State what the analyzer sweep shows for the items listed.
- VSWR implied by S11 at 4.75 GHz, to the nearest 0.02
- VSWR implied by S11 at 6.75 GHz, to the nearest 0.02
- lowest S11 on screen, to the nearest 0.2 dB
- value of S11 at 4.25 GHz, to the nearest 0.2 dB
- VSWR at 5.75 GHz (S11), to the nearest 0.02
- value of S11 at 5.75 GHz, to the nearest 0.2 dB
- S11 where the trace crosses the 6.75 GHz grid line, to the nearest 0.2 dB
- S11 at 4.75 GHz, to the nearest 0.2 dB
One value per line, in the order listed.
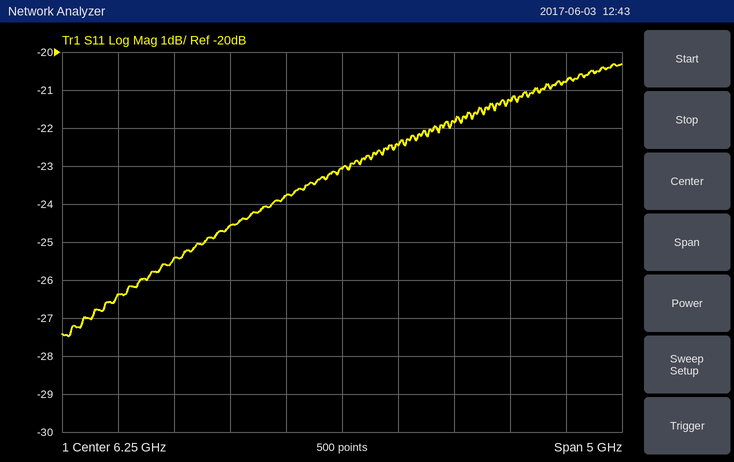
1.12
1.16
-27.4 dB
-26.4 dB
1.14
-23.8 dB
-22.4 dB
-25.4 dB
